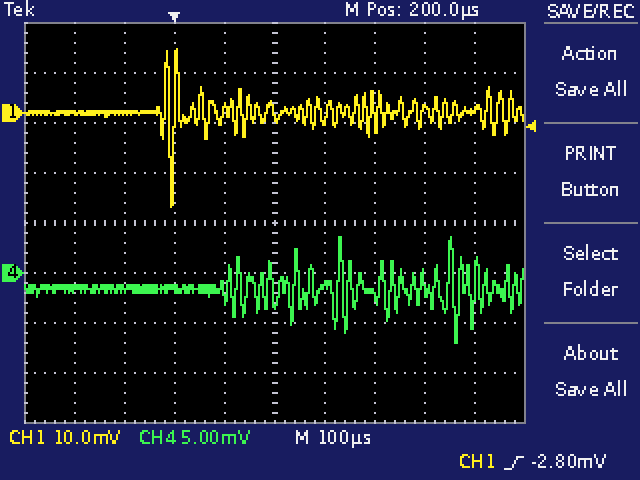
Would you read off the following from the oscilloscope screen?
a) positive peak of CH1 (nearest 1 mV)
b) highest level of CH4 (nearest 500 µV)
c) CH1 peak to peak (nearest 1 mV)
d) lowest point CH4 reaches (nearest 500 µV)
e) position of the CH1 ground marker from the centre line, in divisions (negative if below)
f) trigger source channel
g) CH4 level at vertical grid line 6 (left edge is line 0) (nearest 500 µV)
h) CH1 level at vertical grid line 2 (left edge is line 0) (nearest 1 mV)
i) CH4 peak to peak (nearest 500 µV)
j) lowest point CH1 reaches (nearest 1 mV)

13 mV
3.5 mV
32 mV
-7.0 mV
+2.2 div
CH1
-1.0 mV
0 mV
10.5 mV
-19 mV
